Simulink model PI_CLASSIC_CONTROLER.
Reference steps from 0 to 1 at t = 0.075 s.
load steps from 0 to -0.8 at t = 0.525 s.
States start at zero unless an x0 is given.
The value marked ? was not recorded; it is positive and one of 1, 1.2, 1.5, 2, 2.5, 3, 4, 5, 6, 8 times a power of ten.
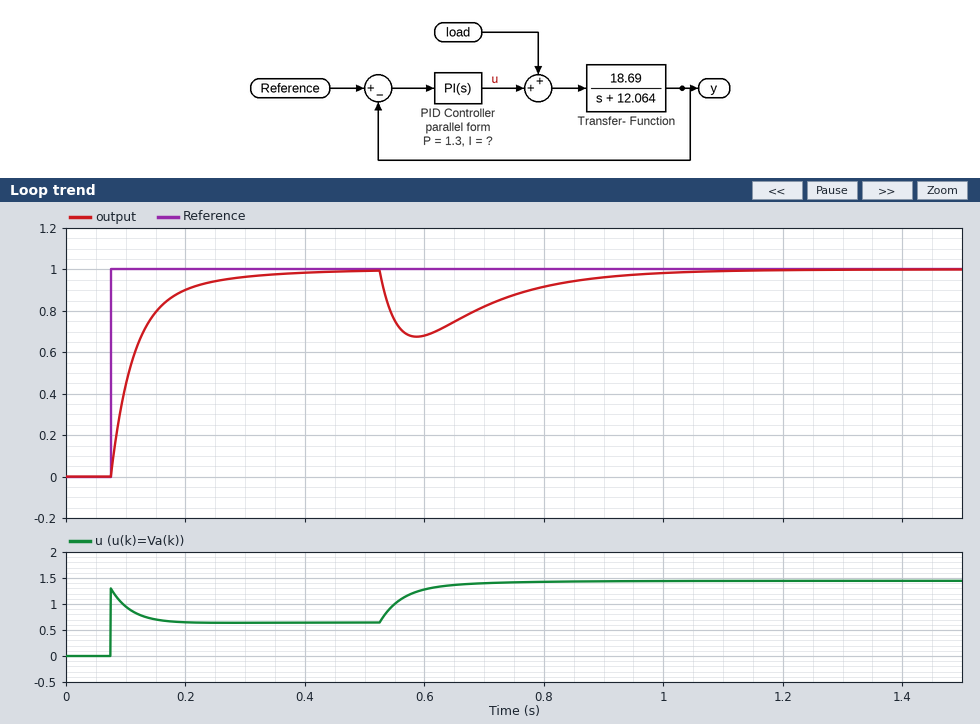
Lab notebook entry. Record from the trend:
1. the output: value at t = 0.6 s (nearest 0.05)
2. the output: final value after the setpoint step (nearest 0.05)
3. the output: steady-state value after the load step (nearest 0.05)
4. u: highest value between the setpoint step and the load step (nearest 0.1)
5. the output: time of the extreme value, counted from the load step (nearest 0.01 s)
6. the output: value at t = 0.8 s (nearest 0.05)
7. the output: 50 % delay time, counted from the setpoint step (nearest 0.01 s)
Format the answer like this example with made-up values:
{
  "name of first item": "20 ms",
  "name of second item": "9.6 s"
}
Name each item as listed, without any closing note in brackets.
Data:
{
  "the output: value at t = 0.6 s": "0.70",
  "the output: final value after the setpoint step": "1.00",
  "the output: steady-state value after the load step": "1.00",
  "u: highest value between the setpoint step and the load step": "1.3",
  "the output: time of the extreme value, counted from the load step": "0.06 s",
  "the output: value at t = 0.8 s": "0.90",
  "the output: 50 % delay time, counted from the setpoint step": "0.03 s"
}
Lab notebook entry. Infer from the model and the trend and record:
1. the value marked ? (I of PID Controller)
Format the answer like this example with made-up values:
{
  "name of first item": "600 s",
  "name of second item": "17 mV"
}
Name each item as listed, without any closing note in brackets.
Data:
{
  "the value marked ?": "12"
}
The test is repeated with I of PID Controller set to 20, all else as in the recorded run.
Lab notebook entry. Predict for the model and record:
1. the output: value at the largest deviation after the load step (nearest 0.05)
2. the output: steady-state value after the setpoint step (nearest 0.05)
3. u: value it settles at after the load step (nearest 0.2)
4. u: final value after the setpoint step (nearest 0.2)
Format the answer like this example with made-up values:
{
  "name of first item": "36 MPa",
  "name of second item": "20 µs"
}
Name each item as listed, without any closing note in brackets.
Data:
{
  "the output: value at the largest deviation after the load step": "0.70",
  "the output: steady-state value after the setpoint step": "1.00",
  "u: value it settles at after the load step": "1.4",
  "u: final value after the setpoint step": "0.6"
}
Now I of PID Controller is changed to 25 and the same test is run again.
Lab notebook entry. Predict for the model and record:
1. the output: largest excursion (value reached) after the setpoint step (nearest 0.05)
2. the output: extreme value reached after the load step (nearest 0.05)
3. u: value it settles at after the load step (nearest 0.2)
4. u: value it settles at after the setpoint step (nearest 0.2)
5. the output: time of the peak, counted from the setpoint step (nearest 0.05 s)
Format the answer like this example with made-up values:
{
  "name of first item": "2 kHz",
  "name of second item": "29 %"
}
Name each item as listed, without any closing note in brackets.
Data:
{
  "the output: largest excursion (value reached) after the setpoint step": "1.05",
  "the output: extreme value reached after the load step": "0.70",
  "u: value it settles at after the load step": "1.4",
  "u: value it settles at after the setpoint step": "0.6",
  "the output: time of the peak, counted from the setpoint step": "0.15 s"
}
